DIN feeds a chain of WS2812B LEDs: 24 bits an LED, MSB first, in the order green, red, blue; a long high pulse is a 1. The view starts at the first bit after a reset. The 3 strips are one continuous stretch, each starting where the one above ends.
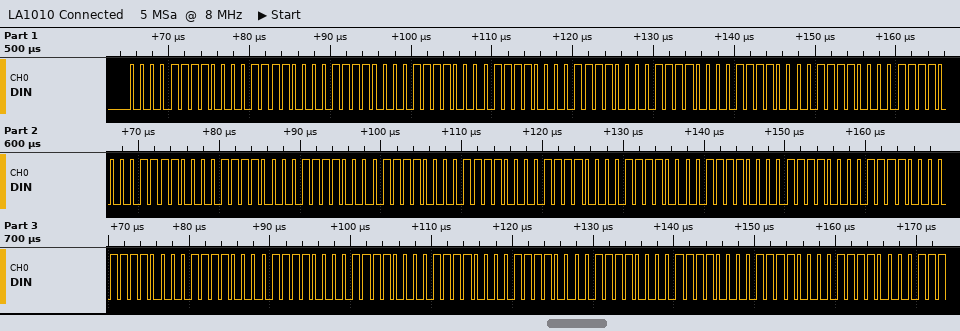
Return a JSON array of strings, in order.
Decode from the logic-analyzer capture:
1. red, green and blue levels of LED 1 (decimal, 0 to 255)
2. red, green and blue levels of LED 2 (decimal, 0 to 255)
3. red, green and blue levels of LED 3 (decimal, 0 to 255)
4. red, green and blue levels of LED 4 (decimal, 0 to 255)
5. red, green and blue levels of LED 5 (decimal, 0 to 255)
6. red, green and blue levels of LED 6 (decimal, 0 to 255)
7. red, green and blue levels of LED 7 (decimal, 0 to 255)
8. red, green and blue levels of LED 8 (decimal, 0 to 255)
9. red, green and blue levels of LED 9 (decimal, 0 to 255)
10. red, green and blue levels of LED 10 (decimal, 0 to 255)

["15, 15, 15", "15, 15, 15", "15, 15, 15", "15, 15, 15", "15, 15, 15", "15, 15, 15", "15, 15, 15", "15, 15, 15", "15, 15, 15", "15, 15, 15"]
